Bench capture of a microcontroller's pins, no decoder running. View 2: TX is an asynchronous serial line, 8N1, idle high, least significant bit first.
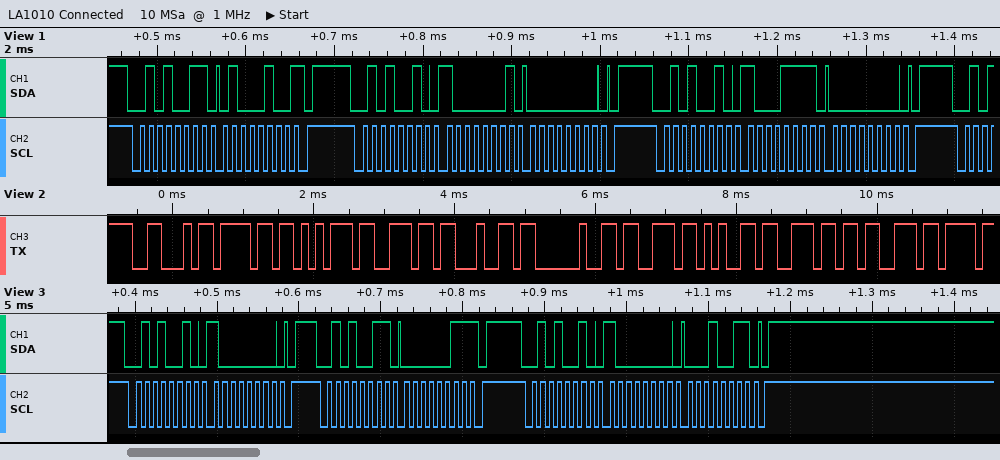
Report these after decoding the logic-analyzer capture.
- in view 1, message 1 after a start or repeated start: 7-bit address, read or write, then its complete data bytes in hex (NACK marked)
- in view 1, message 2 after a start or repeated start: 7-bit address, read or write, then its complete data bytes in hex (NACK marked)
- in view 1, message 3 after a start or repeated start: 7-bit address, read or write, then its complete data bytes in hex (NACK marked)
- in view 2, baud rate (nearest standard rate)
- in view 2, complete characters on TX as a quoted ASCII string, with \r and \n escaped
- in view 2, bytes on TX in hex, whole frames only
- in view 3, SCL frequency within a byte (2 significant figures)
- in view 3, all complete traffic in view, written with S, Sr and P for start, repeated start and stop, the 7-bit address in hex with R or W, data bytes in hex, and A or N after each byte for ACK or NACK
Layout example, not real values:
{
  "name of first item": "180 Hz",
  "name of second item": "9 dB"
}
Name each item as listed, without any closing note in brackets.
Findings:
{
  "in view 1, message 1 after a start or repeated start: 7-bit address, read or write, then its complete data bytes in hex": "0x29 read: 44 NACK",
  "in view 1, message 2 after a start or repeated start: 7-bit address, read or write, then its complete data bytes in hex": "0x29 write: 81 00",
  "in view 1, message 3 after a start or repeated start: 7-bit address, read or write, then its complete data bytes in hex": "0x29 write: 8F 00",
  "in view 2, baud rate": "9600 baud",
  "in view 2, complete characters on TX as a quoted ASCII string, with \\r and \\n escaped": "\"Found sens\"",
  "in view 2, bytes on TX in hex, whole frames only": "46 6F 75 6E 64 20 73 65 6E 73",
  "in view 3, SCL frequency within a byte": "100 kHz",
  "in view 3, all complete traffic in view, written with S, Sr and P for start, repeated start and stop, the 7-bit address in hex with R or W, data bytes in hex, and A or N after each byte for ACK or NACK": "S 29W A 80 A P S 29R A 03 N P S 29W A 80 A 13 A P"
}
